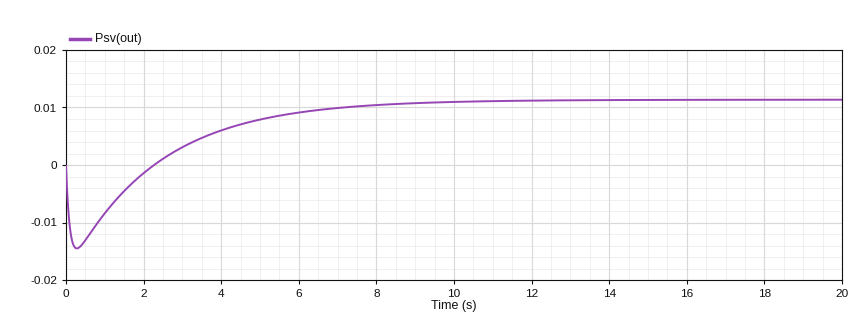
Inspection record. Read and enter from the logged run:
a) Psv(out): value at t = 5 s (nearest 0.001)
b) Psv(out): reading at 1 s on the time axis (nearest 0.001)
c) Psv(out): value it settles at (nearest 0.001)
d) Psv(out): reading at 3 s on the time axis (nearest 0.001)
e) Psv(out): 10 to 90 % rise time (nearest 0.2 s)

0.008
-0.008
0.011
0.003
5.0 s
